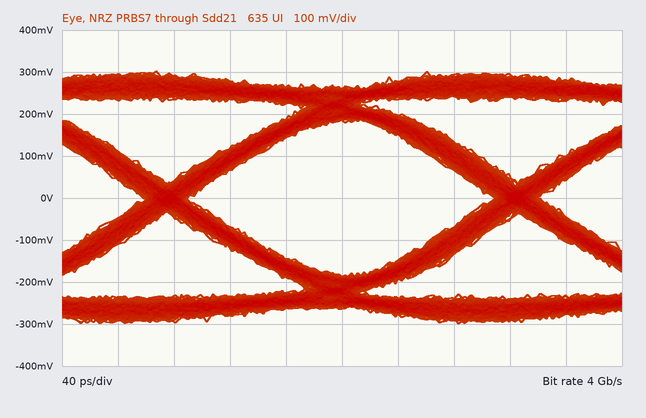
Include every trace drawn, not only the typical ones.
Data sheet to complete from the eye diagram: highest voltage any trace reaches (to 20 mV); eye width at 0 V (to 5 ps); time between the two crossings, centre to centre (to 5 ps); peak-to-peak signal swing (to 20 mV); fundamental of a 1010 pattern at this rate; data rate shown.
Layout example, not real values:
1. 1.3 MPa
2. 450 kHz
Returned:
1. 300 mV
2. 220 ps
3. 250 ps
4. 600 mV
5. 2 GHz
6. 4 Gb/s
